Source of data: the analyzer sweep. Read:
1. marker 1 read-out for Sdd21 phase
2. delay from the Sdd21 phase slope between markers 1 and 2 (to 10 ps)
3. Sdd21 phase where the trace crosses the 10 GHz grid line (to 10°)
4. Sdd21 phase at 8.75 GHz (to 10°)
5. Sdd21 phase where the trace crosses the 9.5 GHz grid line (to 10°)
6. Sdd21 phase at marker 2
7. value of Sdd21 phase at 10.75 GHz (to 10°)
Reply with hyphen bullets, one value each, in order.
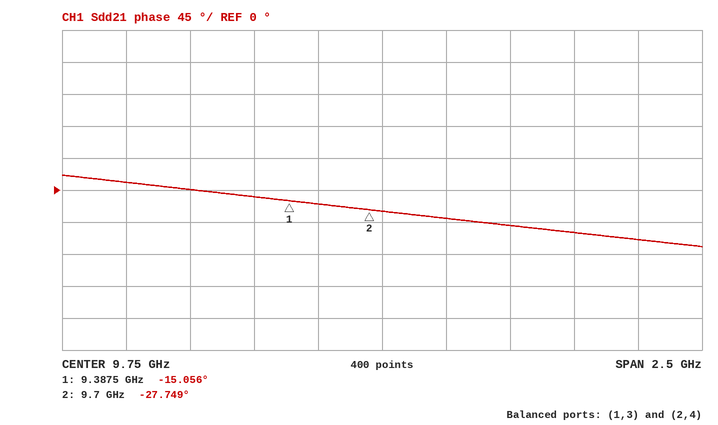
- -15.056°
- 110 ps
- -40°
- 10°
- -20°
- -27.749°
- -70°
